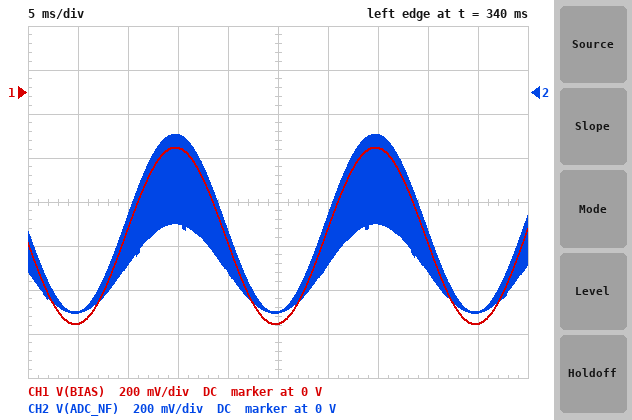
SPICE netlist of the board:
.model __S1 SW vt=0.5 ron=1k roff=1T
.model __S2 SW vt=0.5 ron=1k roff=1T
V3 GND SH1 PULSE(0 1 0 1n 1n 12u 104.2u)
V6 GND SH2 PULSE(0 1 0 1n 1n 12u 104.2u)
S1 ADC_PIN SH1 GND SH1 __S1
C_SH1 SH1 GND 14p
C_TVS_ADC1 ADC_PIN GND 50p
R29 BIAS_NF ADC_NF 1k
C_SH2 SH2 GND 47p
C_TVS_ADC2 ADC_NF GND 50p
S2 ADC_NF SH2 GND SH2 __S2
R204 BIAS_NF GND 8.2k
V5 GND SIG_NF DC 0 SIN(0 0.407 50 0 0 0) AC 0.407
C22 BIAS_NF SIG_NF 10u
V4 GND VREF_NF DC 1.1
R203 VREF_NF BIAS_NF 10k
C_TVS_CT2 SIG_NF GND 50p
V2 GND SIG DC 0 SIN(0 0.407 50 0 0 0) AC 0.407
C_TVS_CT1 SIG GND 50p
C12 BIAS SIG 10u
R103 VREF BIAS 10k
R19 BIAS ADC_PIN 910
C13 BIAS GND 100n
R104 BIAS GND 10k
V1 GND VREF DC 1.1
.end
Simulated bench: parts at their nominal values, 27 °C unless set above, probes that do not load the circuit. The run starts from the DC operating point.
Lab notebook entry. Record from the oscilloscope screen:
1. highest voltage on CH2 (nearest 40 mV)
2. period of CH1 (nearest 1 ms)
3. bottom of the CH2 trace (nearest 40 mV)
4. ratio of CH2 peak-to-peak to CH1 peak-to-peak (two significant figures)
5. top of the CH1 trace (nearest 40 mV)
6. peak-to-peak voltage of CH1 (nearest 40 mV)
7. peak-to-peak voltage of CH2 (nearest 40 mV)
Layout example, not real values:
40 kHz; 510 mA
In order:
-200 mV; 20 ms; -1.00 V; 1.0; -240 mV; 800 mV; 800 mV
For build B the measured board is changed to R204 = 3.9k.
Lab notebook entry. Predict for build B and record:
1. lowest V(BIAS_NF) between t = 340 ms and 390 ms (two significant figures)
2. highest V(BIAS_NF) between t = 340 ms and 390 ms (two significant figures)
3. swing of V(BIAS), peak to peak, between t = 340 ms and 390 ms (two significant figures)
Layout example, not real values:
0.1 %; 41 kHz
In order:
-810 mV; -1.2 mV; 800 mV
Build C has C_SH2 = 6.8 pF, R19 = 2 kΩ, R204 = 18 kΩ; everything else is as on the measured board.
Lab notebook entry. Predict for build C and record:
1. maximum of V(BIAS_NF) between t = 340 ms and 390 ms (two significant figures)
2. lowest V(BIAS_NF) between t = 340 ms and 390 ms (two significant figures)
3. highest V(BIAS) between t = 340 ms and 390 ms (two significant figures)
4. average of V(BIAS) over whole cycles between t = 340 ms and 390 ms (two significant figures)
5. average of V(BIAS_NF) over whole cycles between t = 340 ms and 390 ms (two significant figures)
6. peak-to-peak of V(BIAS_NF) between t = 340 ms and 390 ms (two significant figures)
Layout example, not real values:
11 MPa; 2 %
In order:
-380 mV; -1.2 V; -220 mV; -620 mV; -790 mV; 810 mV
